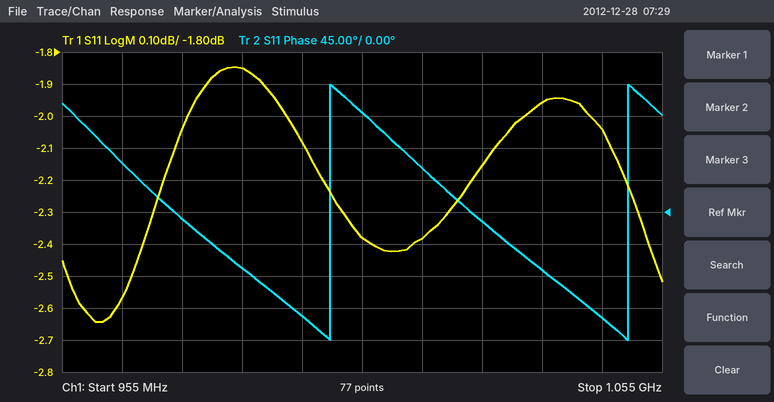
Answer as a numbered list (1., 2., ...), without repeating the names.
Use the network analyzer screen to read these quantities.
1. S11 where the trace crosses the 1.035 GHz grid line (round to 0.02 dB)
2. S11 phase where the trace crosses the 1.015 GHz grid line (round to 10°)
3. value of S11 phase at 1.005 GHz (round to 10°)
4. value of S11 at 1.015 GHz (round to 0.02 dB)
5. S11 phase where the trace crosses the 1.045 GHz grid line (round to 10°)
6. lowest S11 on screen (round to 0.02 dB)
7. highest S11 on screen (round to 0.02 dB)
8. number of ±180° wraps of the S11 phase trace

1. -1.96 dB
2. 60°
3. 140°
4. -2.38 dB
5. -150°
6. -2.64 dB
7. -1.84 dB
8. 2
